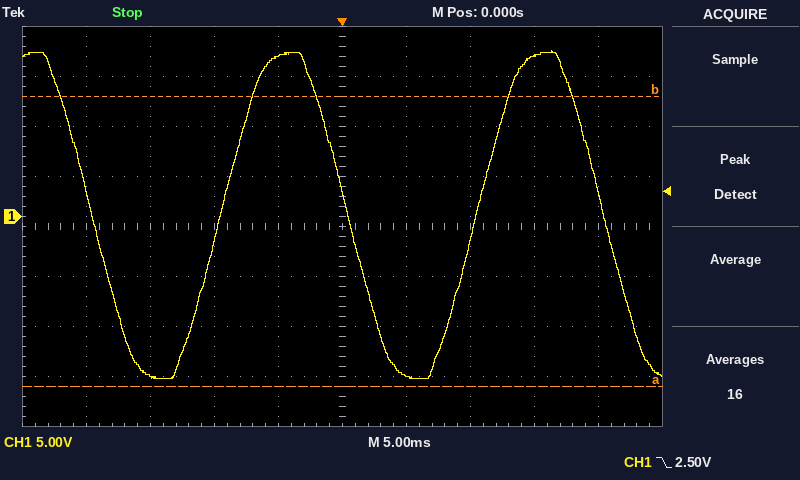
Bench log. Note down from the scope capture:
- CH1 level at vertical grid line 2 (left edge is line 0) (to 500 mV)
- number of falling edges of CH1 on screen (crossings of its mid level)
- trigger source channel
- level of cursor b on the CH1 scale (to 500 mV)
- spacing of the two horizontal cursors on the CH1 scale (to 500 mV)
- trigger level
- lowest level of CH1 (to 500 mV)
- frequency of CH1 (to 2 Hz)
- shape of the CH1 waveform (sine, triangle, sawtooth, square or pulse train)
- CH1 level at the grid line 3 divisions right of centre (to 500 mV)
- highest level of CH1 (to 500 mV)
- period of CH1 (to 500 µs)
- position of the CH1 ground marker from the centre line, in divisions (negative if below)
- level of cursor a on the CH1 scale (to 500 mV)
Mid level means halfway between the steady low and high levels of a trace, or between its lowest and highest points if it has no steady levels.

-16.0 V
3
CH1
12.0 V
29.0 V
2.50 V
-16.0 V
50 Hz
sine
16.0 V
16.5 V
20.0 ms
+0.2 div
-17.0 V
